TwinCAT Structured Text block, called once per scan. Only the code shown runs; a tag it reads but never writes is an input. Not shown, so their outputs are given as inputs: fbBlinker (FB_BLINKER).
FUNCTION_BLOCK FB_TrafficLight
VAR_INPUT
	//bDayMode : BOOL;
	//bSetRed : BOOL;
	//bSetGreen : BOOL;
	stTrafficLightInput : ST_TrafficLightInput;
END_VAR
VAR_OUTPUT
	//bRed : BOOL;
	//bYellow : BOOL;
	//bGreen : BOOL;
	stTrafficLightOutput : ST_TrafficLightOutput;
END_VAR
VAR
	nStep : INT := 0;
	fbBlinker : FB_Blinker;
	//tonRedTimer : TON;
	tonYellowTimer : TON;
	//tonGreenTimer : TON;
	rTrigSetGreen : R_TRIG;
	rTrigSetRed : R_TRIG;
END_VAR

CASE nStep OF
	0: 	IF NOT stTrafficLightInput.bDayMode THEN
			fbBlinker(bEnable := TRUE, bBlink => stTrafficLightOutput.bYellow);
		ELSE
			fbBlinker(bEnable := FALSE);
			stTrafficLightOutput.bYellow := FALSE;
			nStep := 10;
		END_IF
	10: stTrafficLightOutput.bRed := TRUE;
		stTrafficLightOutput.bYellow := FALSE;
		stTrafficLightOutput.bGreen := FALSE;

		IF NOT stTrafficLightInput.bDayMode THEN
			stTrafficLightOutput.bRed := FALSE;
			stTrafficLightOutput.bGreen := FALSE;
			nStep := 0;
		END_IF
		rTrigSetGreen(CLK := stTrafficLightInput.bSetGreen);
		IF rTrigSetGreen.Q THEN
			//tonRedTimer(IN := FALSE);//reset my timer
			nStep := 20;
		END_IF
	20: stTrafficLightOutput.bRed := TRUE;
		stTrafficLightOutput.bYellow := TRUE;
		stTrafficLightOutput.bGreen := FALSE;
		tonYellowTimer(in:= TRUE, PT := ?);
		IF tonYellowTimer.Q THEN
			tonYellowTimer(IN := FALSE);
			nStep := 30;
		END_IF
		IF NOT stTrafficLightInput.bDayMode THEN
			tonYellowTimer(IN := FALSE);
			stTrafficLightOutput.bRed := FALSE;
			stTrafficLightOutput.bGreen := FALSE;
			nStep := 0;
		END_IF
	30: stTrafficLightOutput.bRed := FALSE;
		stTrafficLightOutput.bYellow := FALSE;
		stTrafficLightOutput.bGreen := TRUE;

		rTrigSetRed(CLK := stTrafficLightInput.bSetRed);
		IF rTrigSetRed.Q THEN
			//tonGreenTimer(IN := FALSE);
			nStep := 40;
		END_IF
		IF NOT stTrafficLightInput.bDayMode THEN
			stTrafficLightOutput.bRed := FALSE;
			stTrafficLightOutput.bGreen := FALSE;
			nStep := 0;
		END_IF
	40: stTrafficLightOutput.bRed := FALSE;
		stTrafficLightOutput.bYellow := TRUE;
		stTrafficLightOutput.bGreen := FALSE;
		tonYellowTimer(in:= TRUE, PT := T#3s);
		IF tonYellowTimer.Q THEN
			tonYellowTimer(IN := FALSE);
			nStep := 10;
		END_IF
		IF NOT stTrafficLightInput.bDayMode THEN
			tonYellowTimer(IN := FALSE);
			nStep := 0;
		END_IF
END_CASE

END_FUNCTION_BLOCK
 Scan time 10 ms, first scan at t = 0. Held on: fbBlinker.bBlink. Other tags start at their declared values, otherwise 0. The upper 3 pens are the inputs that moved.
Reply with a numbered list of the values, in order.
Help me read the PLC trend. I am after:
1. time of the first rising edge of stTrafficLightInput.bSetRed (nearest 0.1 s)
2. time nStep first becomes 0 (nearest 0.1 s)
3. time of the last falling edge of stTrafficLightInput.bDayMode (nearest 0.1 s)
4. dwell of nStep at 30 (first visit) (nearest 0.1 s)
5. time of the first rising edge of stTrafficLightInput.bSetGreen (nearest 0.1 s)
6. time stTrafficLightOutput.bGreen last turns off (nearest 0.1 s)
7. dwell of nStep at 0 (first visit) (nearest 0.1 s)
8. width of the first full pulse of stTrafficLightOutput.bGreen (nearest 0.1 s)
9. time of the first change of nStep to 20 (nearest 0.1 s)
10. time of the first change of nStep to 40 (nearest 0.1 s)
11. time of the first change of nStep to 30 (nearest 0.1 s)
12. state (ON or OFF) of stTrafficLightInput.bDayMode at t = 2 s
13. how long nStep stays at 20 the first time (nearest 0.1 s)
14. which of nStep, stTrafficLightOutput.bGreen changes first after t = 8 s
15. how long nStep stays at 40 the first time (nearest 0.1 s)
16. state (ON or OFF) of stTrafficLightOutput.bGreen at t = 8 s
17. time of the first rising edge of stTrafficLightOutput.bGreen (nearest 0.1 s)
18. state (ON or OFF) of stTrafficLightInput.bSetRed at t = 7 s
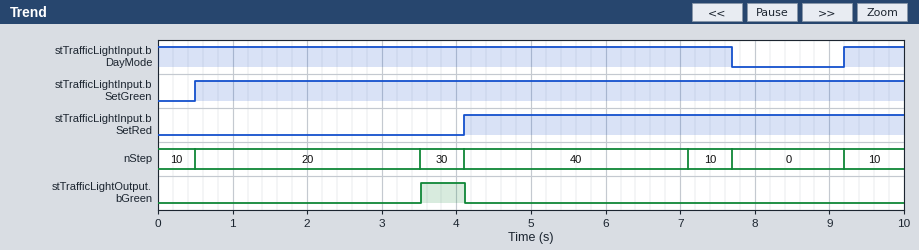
1. 4.1 s
2. 7.7 s
3. 7.7 s
4. 0.6 s
5. 0.5 s
6. 4.1 s
7. 1.5 s
8. 0.6 s
9. 0.5 s
10. 4.1 s
11. 3.5 s
12. ON
13. 3.0 s
14. nStep
15. 3.0 s
16. OFF
17. 3.5 s
18. ON
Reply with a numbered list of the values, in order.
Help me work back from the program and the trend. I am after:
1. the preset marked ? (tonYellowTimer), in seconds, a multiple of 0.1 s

1. 3.0 s
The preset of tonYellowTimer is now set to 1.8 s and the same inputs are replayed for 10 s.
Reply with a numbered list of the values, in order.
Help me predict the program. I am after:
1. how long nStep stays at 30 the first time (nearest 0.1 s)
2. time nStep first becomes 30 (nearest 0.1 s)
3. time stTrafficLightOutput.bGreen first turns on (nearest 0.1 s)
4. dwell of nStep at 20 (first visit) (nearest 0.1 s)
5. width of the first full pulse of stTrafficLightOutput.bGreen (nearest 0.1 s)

1. 1.8 s
2. 2.3 s
3. 2.3 s
4. 1.8 s
5. 1.8 s
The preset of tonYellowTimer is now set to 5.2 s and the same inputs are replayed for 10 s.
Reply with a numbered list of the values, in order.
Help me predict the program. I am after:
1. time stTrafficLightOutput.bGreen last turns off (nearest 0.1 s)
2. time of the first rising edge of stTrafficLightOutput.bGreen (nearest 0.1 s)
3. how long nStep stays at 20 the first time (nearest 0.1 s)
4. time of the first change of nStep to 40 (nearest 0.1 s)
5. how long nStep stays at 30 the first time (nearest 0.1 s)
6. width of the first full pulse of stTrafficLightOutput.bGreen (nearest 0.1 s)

1. 5.7 s
2. 5.7 s
3. 5.2 s
4. 5.7 s
5. 0.0 s
6. 0.0 s
